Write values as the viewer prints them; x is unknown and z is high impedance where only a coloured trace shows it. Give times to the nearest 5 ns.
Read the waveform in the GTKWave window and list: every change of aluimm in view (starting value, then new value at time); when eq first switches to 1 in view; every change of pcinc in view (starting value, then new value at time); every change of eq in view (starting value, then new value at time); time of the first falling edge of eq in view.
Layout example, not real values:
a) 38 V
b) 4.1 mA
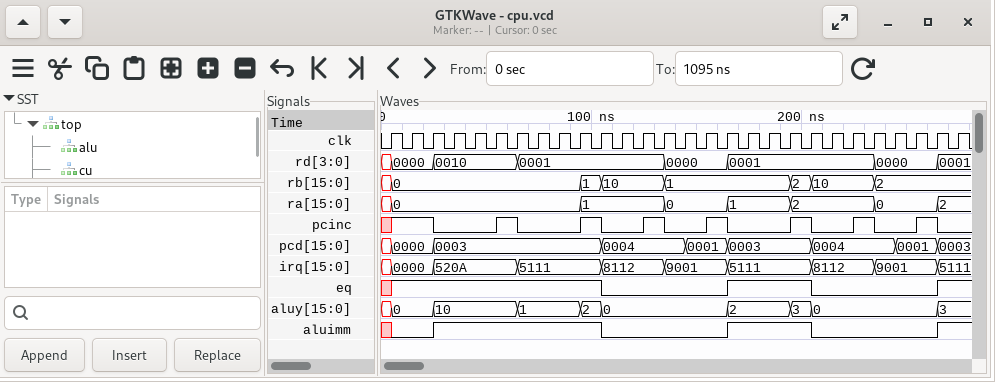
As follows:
a) x, 0 at 5 ns, 1 at 25 ns, 0 at 105 ns, 1 at 165 ns, 0 at 205 ns, 1 at 265 ns
b) 5 ns
c) x, 1 at 5 ns, 0 at 25 ns, 1 at 55 ns, 0 at 65 ns, 1 at 95 ns, 0 at 105 ns, 1 at 125 ns, 0 at 135 ns, 1 at 155 ns, 0 at 165 ns, 1 at 195 ns, 0 at 205 ns, 1 at 225 ns, 0 at 235 ns, 1 at 255 ns, 0 at 265 ns
d) x, 1 at 5 ns, 0 at 105 ns, 1 at 165 ns, 0 at 205 ns, 1 at 265 ns
e) 105 ns
